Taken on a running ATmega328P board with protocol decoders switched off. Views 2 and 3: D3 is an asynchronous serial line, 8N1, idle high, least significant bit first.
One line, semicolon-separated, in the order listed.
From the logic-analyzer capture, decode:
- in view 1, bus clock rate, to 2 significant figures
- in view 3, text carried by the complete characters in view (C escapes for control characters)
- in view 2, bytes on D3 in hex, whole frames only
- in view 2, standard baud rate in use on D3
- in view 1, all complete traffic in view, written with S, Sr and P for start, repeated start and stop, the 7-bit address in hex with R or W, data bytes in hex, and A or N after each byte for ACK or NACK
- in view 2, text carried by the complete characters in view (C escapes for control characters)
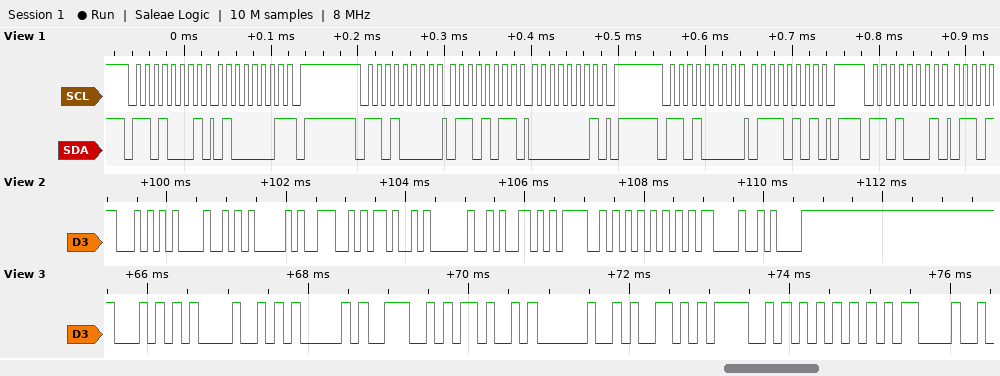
100 kHz; "THANK YOU\r"; 54 48 41 4E 4B 20 59 4F 55 0D 0A; 9600 baud; S 68R A 41 N P S 68W A 6B A 01 A P S 68W A 75 A P S 68R A; "THANK YOU\r\n"
